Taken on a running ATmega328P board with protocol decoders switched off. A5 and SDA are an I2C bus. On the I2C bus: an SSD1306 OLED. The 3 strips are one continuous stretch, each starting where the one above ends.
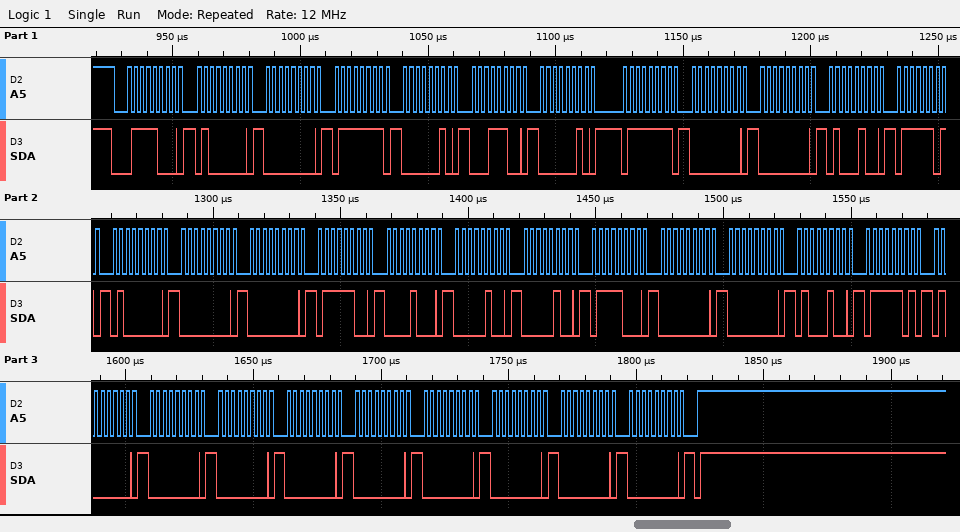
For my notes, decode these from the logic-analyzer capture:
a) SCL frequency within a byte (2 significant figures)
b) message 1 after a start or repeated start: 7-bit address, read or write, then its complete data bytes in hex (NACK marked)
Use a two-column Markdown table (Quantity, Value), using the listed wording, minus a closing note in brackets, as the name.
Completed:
| Quantity | Value |
|---|---|
| SCL frequency within a byte | 400 kHz |
| message 1 after a start or repeated start: 7-bit address, read or write, then its complete data bytes in hex | 0x3C write: 40 00 7F 02 1C 02 7F 00 00 44 7D 40 00 00 7C 08 04 04 78 00 00 44 7D 40 00 00 00 00 00 00 00 00 |
